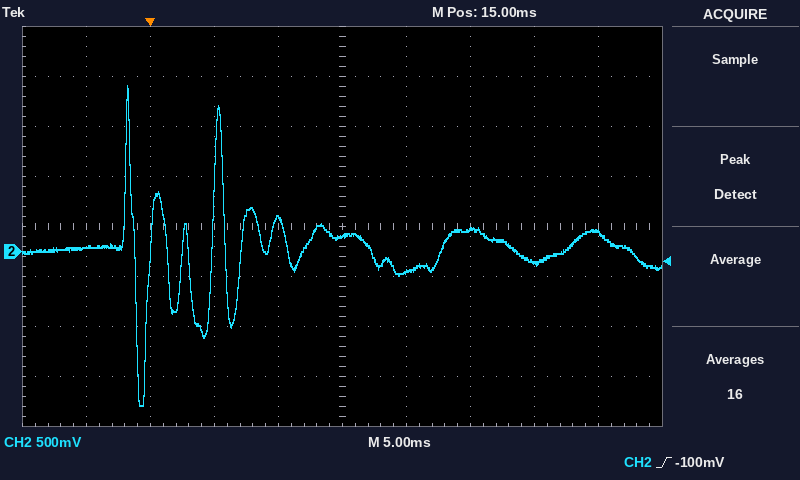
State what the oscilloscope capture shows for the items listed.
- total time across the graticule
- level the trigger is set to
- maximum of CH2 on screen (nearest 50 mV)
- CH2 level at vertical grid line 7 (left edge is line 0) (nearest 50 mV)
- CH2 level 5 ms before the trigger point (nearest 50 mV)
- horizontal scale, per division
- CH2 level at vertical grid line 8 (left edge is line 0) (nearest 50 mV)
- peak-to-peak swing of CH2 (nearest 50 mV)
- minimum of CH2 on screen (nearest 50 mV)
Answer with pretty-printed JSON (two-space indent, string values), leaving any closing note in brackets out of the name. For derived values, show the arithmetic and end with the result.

{
  "total time across the graticule": "50 ms",
  "level the trigger is set to": "-100 mV",
  "maximum of CH2 on screen": "1.65 V",
  "CH2 level at vertical grid line 7 (left edge is line 0)": "200 mV",
  "CH2 level 5 ms before the trigger point": "50 mV",
  "horizontal scale, per division": "5 ms",
  "CH2 level at vertical grid line 8 (left edge is line 0)": "-100 mV",
  "peak-to-peak swing of CH2": "1.65 V − (-1.55 V) = 3.20 V",
  "minimum of CH2 on screen": "-1.55 V"
}
